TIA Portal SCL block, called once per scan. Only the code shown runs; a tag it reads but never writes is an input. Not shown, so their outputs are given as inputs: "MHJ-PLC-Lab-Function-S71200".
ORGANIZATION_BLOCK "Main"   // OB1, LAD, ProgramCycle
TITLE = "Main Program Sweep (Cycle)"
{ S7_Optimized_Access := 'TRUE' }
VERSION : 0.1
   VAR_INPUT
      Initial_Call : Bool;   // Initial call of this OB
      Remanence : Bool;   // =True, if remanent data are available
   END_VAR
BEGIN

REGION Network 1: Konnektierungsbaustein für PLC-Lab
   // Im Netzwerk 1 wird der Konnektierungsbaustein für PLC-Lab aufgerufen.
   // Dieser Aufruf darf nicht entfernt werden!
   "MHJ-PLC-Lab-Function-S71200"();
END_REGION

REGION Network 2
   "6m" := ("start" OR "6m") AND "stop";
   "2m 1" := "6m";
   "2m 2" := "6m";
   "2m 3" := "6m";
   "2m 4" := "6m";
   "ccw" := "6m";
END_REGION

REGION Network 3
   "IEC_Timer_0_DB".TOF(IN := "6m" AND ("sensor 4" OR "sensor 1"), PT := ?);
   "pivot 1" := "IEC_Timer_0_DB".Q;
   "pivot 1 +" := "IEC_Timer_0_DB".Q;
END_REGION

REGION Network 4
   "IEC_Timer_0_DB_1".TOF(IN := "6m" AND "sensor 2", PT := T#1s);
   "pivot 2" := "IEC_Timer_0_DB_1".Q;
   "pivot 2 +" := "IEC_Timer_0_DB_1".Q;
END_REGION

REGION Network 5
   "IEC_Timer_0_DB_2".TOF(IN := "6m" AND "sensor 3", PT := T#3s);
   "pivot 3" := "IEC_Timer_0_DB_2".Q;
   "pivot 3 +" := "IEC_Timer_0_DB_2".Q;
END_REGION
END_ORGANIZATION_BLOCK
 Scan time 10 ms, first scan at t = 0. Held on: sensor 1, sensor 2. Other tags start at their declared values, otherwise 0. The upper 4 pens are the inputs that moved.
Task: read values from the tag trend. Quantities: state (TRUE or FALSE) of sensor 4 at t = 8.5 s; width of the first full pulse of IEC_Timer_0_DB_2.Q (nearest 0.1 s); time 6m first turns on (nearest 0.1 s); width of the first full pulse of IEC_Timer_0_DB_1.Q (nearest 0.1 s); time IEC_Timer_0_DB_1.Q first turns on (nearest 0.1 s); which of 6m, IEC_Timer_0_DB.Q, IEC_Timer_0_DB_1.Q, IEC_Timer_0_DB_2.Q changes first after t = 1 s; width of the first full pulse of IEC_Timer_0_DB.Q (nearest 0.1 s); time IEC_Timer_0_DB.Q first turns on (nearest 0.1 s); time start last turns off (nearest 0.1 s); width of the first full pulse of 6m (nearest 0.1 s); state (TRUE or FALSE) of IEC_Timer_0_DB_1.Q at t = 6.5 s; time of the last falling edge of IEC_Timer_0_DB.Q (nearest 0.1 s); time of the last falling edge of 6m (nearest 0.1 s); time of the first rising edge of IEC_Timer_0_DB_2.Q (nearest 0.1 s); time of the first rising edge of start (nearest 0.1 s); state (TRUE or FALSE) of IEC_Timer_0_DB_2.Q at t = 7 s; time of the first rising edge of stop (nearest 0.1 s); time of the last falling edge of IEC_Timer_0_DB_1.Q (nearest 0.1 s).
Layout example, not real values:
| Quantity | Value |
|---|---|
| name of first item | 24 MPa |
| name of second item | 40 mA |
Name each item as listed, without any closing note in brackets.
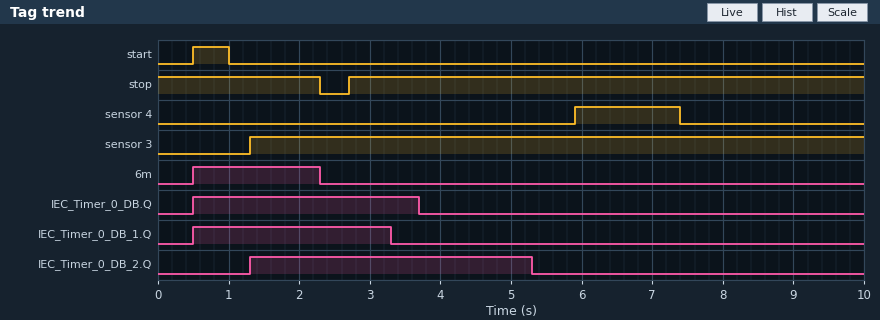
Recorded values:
| Quantity | Value |
|---|---|
| state (TRUE or FALSE) of sensor 4 at t = 8.5 s | FALSE |
| width of the first full pulse of IEC_Timer_0_DB_2.Q | 4.0 s |
| time 6m first turns on | 0.5 s |
| width of the first full pulse of IEC_Timer_0_DB_1.Q | 2.8 s |
| time IEC_Timer_0_DB_1.Q first turns on | 0.5 s |
| which of 6m, IEC_Timer_0_DB.Q, IEC_Timer_0_DB_1.Q, IEC_Timer_0_DB_2.Q changes first after t = 1 s | IEC_Timer_0_DB_2.Q |
| width of the first full pulse of IEC_Timer_0_DB.Q | 3.2 s |
| time IEC_Timer_0_DB.Q first turns on | 0.5 s |
| time start last turns off | 1.0 s |
| width of the first full pulse of 6m | 1.8 s |
| state (TRUE or FALSE) of IEC_Timer_0_DB_1.Q at t = 6.5 s | FALSE |
| time of the last falling edge of IEC_Timer_0_DB.Q | 3.7 s |
| time of the last falling edge of 6m | 2.3 s |
| time of the first rising edge of IEC_Timer_0_DB_2.Q | 1.3 s |
| time of the first rising edge of start | 0.5 s |
| state (TRUE or FALSE) of IEC_Timer_0_DB_2.Q at t = 7 s | FALSE |
| time of the first rising edge of stop | 2.7 s |
| time of the last falling edge of IEC_Timer_0_DB_1.Q | 3.3 s |
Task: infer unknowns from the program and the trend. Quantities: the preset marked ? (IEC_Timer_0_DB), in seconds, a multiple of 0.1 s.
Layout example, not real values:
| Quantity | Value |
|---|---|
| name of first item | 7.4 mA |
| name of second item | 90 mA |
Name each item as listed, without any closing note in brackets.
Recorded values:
| Quantity | Value |
|---|---|
| the preset marked ? (IEC_Timer_0_DB), in seconds, a multiple of 0.1 s | 1.4 s |
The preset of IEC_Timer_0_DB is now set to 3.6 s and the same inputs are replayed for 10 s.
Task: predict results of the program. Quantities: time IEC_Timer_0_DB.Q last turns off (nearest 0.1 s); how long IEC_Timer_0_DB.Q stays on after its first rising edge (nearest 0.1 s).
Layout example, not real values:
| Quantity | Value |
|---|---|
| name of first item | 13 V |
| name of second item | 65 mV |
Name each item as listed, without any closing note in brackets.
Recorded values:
| Quantity | Value |
|---|---|
| time IEC_Timer_0_DB.Q last turns off | 5.9 s |
| how long IEC_Timer_0_DB.Q stays on after its first rising edge | 5.4 s |
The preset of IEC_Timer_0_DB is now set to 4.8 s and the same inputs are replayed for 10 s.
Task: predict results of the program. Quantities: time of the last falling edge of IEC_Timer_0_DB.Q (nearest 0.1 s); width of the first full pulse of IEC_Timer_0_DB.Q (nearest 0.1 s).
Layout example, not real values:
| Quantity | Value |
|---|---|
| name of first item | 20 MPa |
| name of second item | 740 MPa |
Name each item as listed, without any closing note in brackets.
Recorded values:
| Quantity | Value |
|---|---|
| time of the last falling edge of IEC_Timer_0_DB.Q | 7.1 s |
| width of the first full pulse of IEC_Timer_0_DB.Q | 6.6 s |
